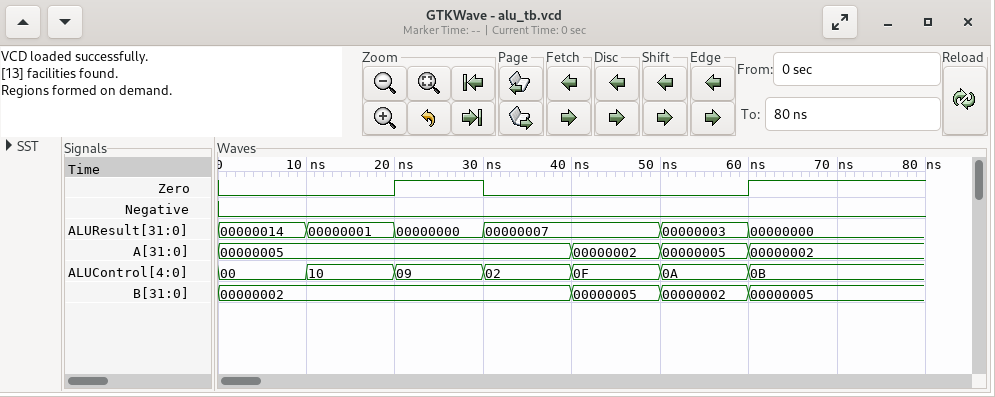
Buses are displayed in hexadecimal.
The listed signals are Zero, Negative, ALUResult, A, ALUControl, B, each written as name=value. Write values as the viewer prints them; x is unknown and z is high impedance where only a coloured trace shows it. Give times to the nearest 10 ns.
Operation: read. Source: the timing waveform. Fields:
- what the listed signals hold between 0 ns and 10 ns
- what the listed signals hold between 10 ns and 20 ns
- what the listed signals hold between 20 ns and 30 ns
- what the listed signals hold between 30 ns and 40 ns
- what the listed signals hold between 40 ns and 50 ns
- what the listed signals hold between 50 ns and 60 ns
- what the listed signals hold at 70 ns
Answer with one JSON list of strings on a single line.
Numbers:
["Zero=0, Negative=0, ALUResult=00000014, A=00000005, ALUControl=00, B=00000002", "Zero=0, Negative=0, ALUResult=00000001, A=00000005, ALUControl=10, B=00000002", "Zero=1, Negative=0, ALUResult=00000000, A=00000005, ALUControl=09, B=00000002", "Zero=0, Negative=0, ALUResult=00000007, A=00000005, ALUControl=02, B=00000002", "Zero=0, Negative=0, ALUResult=00000007, A=00000002, ALUControl=0F, B=00000005", "Zero=0, Negative=0, ALUResult=00000003, A=00000005, ALUControl=0A, B=00000002", "Zero=1, Negative=0, ALUResult=00000000, A=00000002, ALUControl=0B, B=00000005"]
